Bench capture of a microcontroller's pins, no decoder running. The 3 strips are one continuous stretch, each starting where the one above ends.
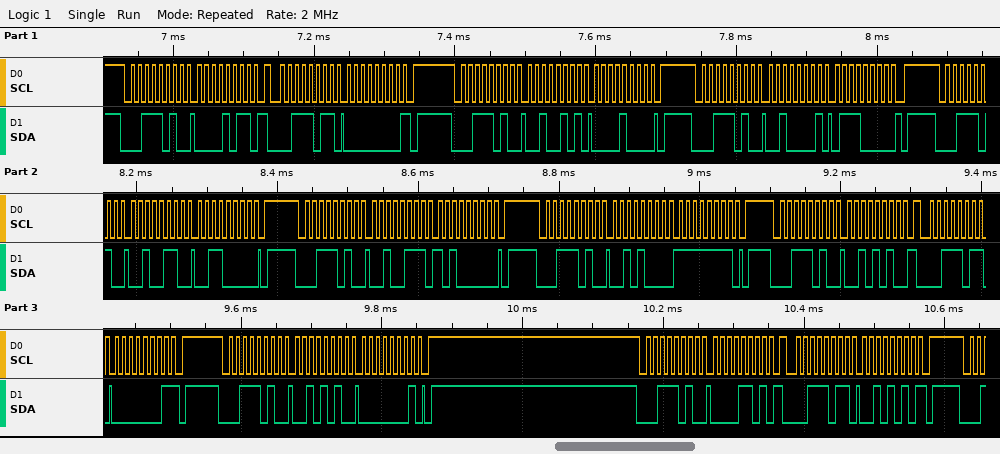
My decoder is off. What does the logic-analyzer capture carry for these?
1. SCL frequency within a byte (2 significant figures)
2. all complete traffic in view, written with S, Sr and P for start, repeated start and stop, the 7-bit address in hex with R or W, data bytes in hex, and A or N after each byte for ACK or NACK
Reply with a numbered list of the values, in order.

1. 100 kHz
2. S 1DW A 0B A Sr 1DR A 00 N P S 1DW A 25 A 08 A P S 1DW A 21 A 70 A P S 1DW A 26 A 30 A P S 1DW A 27 A A0 A P S 1DW A 28 A FF A P S 1DW A 2A A Sr 1DR A 01 N P S 1DW A 2A A 01 A P S 1DW A 0D A Sr 1DR A 2A N P
